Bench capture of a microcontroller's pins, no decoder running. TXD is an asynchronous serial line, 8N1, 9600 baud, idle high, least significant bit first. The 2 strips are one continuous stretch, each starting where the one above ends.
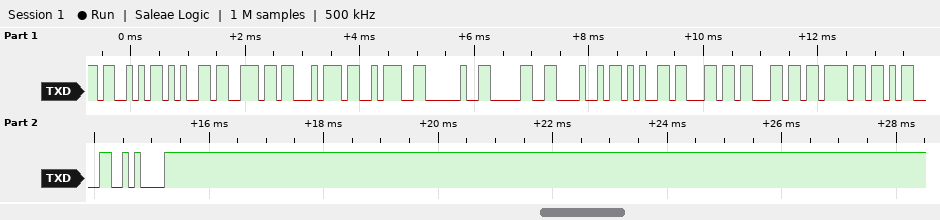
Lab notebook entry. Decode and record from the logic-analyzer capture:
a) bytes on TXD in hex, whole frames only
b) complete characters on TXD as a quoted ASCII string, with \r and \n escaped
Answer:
53 65 6E 74 3A 20 30 48 65 6C 6C 6F 0D 0A
"Sent: 0Hello\r\n"
